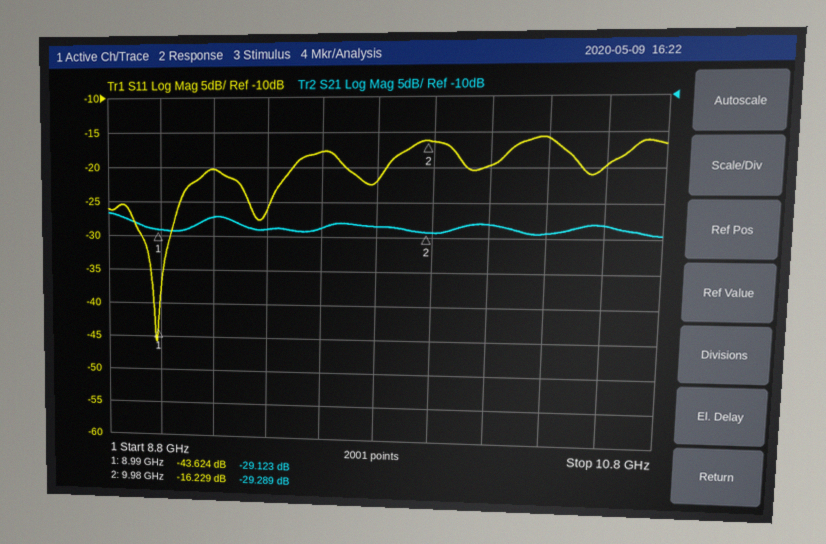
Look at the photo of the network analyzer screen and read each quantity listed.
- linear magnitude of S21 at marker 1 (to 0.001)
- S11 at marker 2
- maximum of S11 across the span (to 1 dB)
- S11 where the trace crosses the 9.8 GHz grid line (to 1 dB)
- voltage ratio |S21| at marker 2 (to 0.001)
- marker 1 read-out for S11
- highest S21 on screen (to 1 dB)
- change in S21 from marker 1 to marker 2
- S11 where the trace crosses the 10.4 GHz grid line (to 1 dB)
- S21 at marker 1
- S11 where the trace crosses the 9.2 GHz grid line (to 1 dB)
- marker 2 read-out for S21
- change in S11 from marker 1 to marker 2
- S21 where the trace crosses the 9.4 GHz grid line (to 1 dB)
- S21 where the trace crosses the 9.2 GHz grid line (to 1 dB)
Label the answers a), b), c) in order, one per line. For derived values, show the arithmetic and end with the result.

a) 10^(-29.123/20) ≈ 0.035
b) -16.229 dB
c) -16 dB
d) -22 dB
e) 10^(-29.289/20) ≈ 0.034
f) -43.624 dB
g) -27 dB
h) -29.289 − (-29.123) = -0.166 dB
i) -16 dB
j) -29.123 dB
k) -20 dB
l) -29.289 dB
m) -16.229 − (-43.624) = 27.395 dB
n) -29 dB
o) -27 dB
